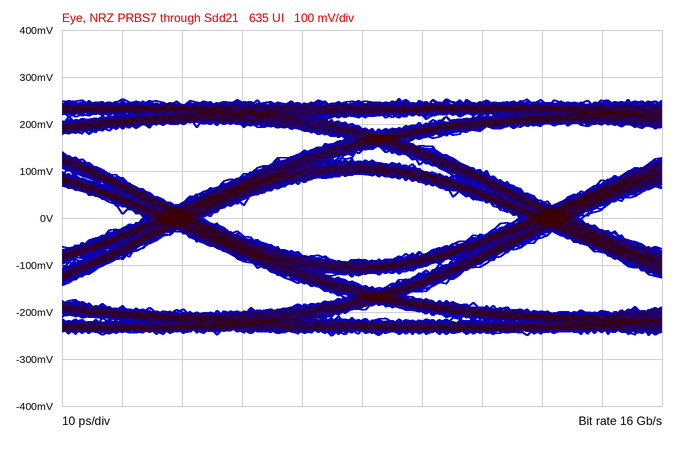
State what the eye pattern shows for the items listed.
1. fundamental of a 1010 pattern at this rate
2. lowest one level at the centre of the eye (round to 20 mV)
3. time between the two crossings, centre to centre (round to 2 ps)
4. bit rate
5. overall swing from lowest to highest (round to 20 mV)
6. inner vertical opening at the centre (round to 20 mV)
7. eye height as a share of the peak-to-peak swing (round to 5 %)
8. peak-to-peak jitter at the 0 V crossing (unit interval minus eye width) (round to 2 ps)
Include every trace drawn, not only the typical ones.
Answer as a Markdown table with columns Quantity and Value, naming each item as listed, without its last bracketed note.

| Quantity | Value |
|---|---|
| fundamental of a 1010 pattern at this rate | 8 GHz |
| lowest one level at the centre of the eye | 100 mV |
| time between the two crossings, centre to centre | 62 ps |
| bit rate | 16 Gb/s |
| overall swing from lowest to highest | 500 mV |
| inner vertical opening at the centre | 180 mV |
| eye height as a share of the peak-to-peak swing | 35 % |
| peak-to-peak jitter at the 0 V crossing (unit interval minus eye width) | 10 ps |
